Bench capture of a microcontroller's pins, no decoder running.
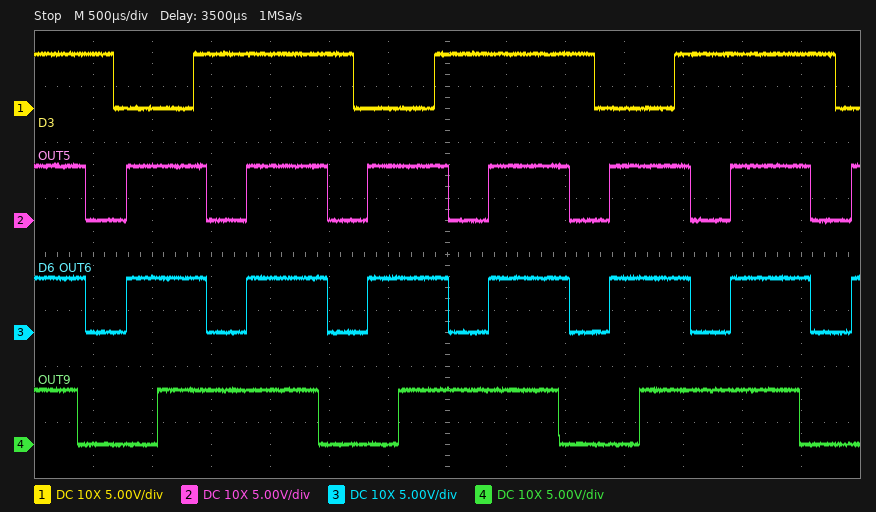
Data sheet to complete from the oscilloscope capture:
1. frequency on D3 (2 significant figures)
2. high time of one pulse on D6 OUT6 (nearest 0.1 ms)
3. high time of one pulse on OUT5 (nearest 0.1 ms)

490 Hz
0.7 ms
0.7 ms
